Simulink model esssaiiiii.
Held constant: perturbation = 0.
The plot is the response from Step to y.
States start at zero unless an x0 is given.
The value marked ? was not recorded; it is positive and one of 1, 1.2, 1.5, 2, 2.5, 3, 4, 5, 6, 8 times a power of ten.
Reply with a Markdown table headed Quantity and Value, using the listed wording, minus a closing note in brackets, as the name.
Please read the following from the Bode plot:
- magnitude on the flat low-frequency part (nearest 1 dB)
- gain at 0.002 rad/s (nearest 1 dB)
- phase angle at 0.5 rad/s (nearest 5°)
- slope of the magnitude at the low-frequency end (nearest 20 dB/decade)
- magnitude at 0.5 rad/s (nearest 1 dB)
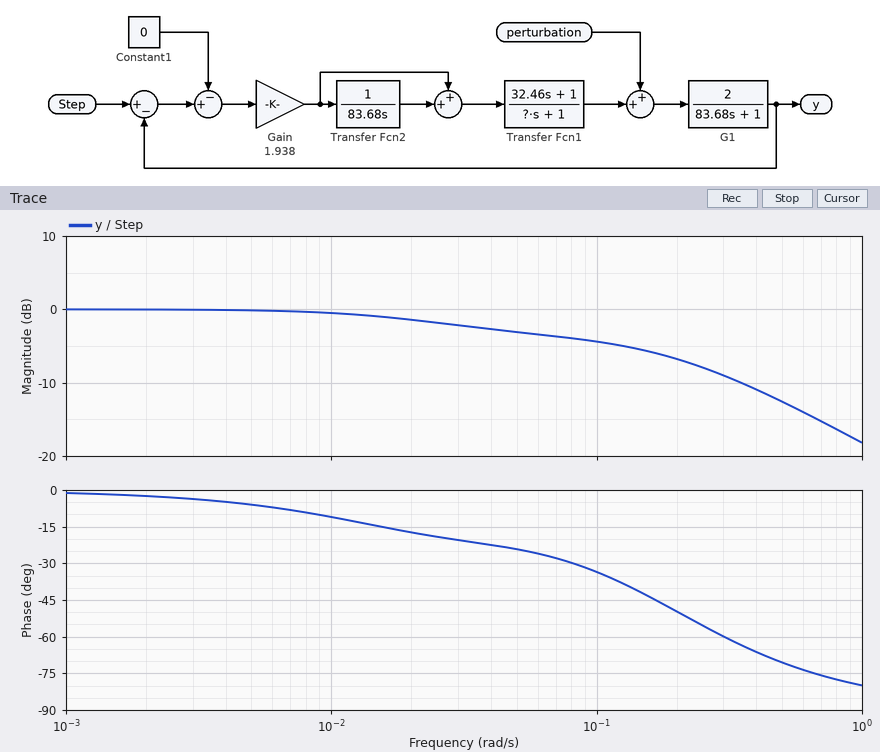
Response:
| Quantity | Value |
|---|---|
| magnitude on the flat low-frequency part | 0 dB |
| gain at 0.002 rad/s | 0 dB |
| phase angle at 0.5 rad/s | -70° |
| slope of the magnitude at the low-frequency end | 0 dB/decade |
| magnitude at 0.5 rad/s | -13 dB |
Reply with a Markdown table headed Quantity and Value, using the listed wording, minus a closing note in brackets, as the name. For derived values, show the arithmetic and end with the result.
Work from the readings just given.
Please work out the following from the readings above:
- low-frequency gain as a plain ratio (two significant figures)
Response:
| Quantity | Value |
|---|---|
| low-frequency gain as a plain ratio | 10^(0 / 20) = 1.0 |
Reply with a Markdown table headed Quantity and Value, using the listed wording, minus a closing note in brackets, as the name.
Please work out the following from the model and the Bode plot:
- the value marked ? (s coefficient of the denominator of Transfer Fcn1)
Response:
| Quantity | Value |
|---|---|
| the value marked ? | 12 |
